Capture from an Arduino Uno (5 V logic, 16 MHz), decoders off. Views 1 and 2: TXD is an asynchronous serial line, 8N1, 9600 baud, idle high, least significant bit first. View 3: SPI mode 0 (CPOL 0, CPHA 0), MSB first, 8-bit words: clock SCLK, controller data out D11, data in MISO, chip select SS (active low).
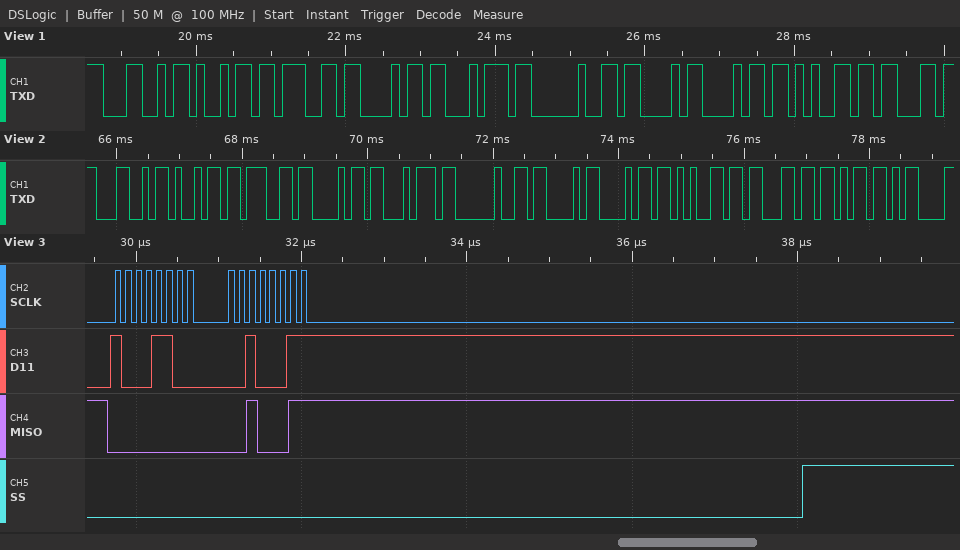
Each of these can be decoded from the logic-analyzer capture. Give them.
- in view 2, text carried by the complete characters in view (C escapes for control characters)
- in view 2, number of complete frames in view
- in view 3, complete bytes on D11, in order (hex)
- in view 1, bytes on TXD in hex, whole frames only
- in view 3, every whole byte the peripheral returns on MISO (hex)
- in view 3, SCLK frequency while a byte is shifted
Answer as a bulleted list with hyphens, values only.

- "Light Check\r"
- 12
- 8C 23
- 4C 69 67 68 74 20 43 68 65 63
- 00 23
- 8 MHz
